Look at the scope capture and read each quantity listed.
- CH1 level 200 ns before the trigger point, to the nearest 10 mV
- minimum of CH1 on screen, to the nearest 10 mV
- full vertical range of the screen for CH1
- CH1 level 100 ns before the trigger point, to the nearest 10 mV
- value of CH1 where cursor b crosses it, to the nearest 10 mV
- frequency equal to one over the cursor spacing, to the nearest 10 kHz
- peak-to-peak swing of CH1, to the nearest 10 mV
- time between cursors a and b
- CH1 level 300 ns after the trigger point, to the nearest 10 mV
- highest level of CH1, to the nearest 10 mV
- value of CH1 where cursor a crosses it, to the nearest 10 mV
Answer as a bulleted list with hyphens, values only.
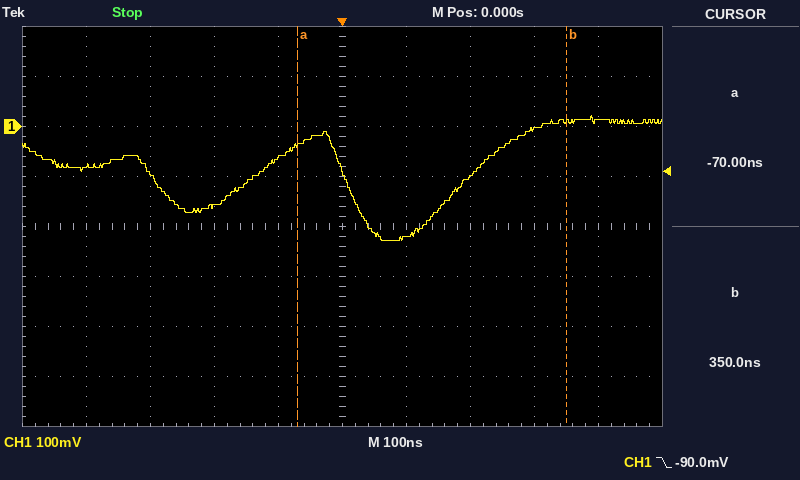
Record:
- -160 mV
- -230 mV
- 800 mV
- -60 mV
- 10 mV
- 2.38 MHz
- 250 mV
- 420 ns
- -10 mV
- 20 mV
- -40 mV
